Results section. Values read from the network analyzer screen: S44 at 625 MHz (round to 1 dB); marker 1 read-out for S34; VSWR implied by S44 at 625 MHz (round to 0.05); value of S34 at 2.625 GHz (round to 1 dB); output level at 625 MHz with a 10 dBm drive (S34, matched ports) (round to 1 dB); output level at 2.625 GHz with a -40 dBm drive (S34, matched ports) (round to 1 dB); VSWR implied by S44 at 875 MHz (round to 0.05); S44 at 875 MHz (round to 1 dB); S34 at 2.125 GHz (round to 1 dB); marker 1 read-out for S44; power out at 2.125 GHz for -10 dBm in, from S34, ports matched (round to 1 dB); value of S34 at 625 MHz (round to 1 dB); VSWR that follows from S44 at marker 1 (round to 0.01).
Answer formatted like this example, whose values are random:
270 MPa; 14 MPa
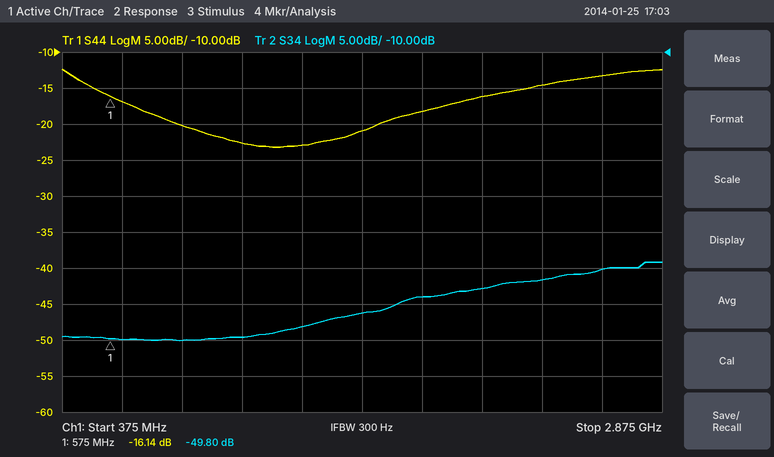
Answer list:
-17 dB; -49.80 dB; 1.35; -40 dB; -40 dBm; -80 dBm; 1.20; -20 dB; -43 dB; -16.14 dB; -53 dBm; -50 dB; 1.37
